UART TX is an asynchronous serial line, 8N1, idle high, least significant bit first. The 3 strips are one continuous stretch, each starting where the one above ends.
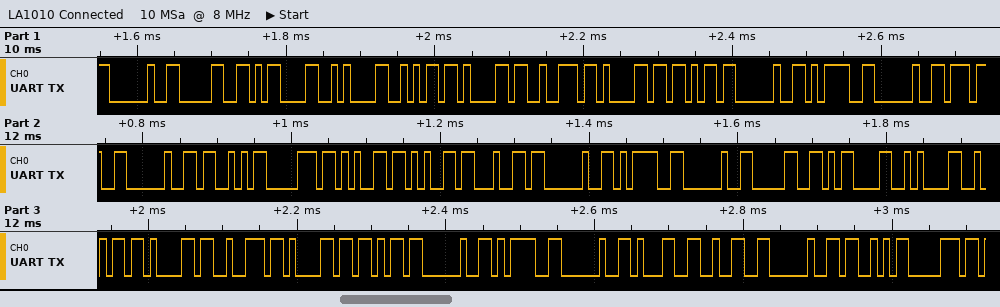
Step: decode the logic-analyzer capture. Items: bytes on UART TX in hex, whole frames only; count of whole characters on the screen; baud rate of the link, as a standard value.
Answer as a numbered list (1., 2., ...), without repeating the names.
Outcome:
1. 20 30 0D 0A 6A 61 72 61 6B 20 3D 20 37 20 53 70 65 65 64 20 3D 20 30 0D 0A 6A 61 72 61 6B 20 3D 20 31 32 20 53 70
2. 38
3. 115200 baud
